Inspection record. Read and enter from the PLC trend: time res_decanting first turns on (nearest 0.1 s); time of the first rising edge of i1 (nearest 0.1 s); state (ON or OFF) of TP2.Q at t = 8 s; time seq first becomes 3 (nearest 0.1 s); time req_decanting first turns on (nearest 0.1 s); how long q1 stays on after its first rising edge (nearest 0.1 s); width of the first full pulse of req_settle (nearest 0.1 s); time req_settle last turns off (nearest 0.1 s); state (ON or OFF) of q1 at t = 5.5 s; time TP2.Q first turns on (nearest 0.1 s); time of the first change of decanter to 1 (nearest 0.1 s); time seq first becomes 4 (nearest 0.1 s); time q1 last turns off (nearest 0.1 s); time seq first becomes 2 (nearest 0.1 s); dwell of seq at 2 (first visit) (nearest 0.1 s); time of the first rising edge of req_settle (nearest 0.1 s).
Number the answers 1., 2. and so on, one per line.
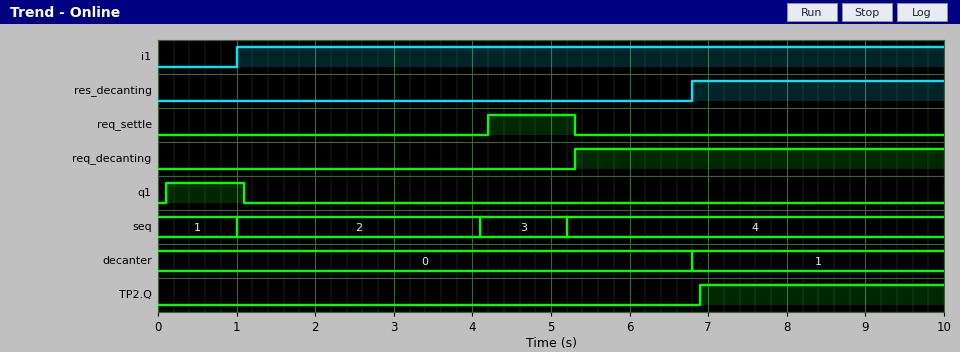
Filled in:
1. 6.8 s
2. 1.0 s
3. ON
4. 4.1 s
5. 5.3 s
6. 1.0 s
7. 1.1 s
8. 5.3 s
9. OFF
10. 6.9 s
11. 6.8 s
12. 5.2 s
13. 1.1 s
14. 1.0 s
15. 3.1 s
16. 4.2 s
